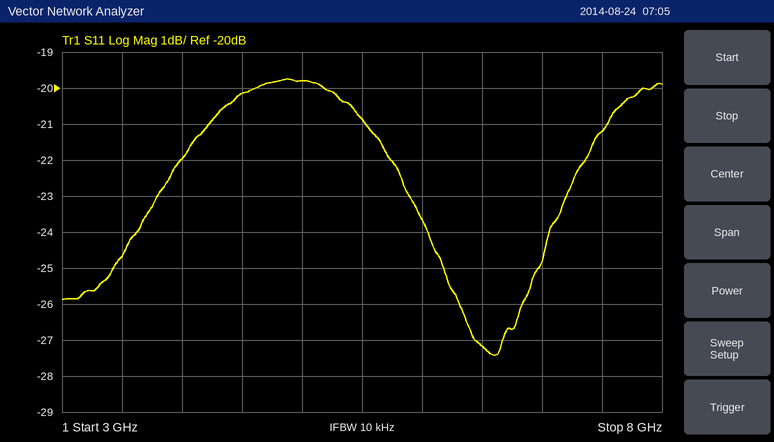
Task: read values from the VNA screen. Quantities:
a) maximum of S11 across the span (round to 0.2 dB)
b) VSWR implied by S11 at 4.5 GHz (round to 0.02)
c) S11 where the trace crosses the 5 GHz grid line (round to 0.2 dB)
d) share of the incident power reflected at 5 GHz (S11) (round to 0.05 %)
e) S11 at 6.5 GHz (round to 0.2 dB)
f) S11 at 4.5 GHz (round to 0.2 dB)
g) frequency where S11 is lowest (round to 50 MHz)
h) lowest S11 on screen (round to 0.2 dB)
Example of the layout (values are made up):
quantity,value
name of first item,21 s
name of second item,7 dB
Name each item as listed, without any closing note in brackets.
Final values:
quantity,value
maximum of S11 across the span,-19.8 dB
VSWR implied by S11 at 4.5 GHz,1.22
S11 where the trace crosses the 5 GHz grid line,-19.8 dB
share of the incident power reflected at 5 GHz (S11),1.05 %
S11 at 6.5 GHz,-27.2 dB
S11 at 4.5 GHz,-20.2 dB
frequency where S11 is lowest,6.60 GHz
lowest S11 on screen,-27.4 dB
